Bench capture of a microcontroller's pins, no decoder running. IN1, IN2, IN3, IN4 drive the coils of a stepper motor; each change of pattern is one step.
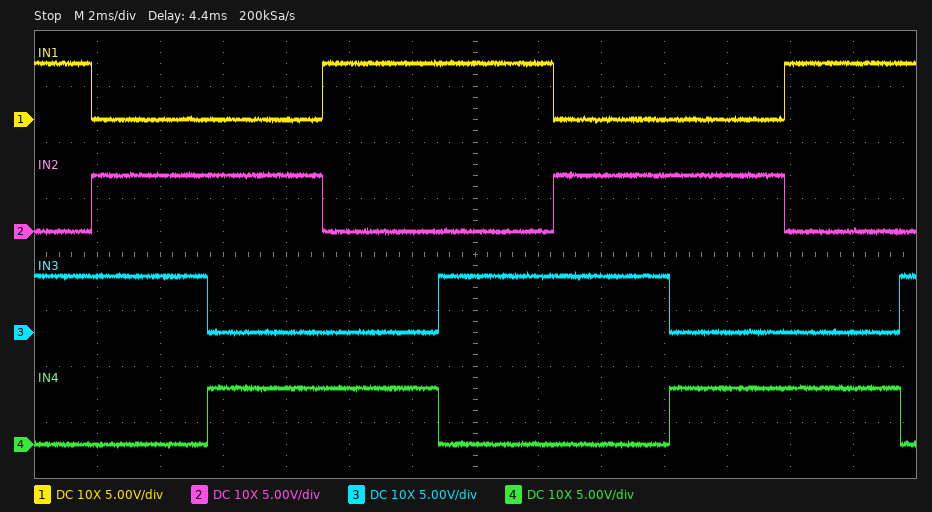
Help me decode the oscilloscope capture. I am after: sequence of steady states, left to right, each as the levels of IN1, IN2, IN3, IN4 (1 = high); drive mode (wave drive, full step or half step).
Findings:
1010 0110 0101 1001 1010 0110 0101 1001 1010
full step
